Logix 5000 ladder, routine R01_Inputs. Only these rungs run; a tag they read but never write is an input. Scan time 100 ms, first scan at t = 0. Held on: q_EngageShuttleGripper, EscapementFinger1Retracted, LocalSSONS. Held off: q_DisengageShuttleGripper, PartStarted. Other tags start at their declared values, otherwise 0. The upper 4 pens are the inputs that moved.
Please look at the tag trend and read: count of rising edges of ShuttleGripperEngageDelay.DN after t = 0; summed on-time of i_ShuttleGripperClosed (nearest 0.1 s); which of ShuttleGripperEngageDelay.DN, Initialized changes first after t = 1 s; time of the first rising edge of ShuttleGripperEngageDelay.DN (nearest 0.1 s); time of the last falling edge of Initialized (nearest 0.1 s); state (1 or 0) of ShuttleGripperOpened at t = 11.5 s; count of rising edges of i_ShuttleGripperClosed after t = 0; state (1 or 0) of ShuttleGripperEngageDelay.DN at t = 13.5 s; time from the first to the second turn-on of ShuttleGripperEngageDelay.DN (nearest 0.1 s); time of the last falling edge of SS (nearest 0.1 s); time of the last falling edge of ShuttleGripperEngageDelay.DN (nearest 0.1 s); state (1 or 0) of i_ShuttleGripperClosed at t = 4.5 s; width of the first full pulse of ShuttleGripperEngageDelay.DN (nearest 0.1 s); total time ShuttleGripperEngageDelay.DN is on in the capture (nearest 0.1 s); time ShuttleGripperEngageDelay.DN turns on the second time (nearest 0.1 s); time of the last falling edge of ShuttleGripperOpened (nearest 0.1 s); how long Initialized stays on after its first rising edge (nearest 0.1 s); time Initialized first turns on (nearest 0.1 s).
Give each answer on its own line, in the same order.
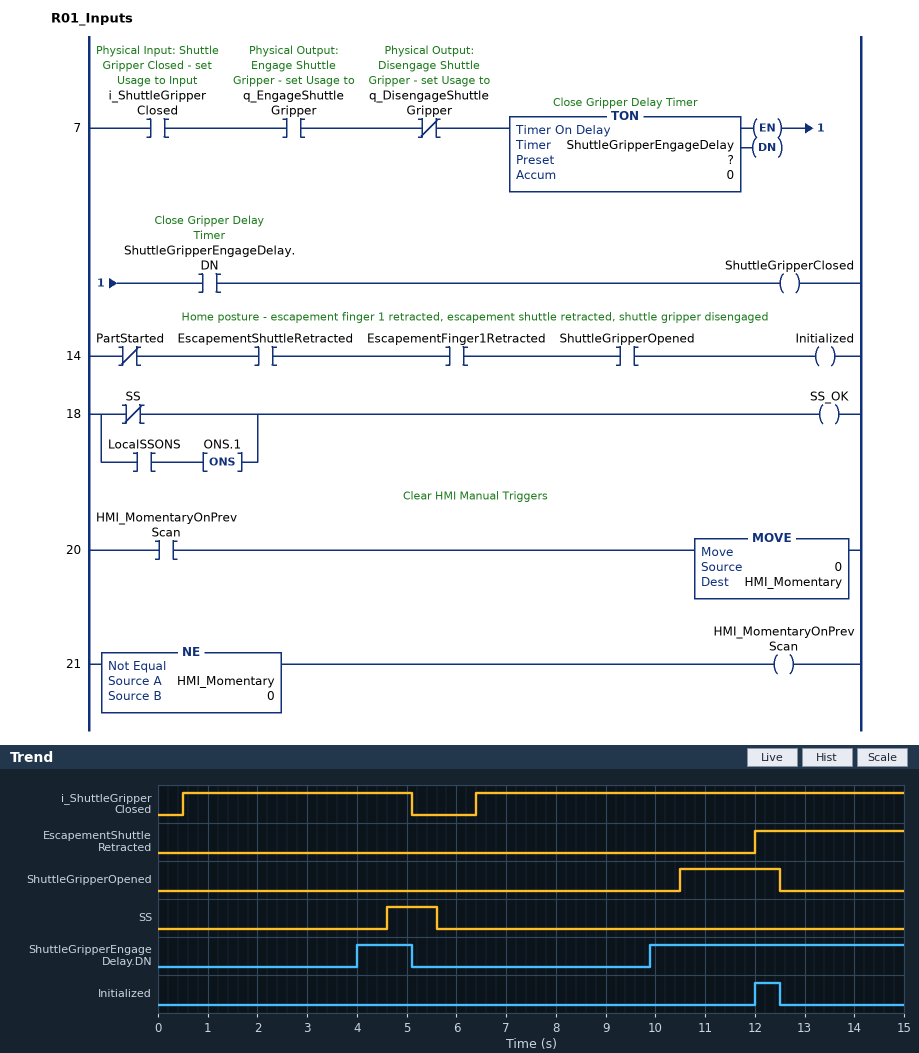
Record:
2
13.2 s
ShuttleGripperEngageDelay.DN
4.0 s
12.5 s
1
2
1
5.9 s
5.6 s
5.1 s
1
1.1 s
6.2 s
9.9 s
12.5 s
0.5 s
12.0 s
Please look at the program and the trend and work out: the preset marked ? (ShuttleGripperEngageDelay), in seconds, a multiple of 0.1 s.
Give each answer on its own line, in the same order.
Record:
3.5 s
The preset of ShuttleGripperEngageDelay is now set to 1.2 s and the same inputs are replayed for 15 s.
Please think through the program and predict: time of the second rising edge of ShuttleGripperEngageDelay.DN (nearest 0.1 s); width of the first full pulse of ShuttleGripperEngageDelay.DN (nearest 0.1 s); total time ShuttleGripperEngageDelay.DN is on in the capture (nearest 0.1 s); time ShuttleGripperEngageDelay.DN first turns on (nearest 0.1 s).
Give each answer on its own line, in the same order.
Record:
7.6 s
3.4 s
10.8 s
1.7 s
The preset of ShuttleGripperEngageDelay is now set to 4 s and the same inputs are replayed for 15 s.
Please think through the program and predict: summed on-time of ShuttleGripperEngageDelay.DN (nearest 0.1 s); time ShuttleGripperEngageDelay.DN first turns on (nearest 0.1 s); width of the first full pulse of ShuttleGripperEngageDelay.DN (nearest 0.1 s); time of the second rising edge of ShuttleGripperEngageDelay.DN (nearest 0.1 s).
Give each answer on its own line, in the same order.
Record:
5.2 s
4.5 s
0.6 s
10.4 s
